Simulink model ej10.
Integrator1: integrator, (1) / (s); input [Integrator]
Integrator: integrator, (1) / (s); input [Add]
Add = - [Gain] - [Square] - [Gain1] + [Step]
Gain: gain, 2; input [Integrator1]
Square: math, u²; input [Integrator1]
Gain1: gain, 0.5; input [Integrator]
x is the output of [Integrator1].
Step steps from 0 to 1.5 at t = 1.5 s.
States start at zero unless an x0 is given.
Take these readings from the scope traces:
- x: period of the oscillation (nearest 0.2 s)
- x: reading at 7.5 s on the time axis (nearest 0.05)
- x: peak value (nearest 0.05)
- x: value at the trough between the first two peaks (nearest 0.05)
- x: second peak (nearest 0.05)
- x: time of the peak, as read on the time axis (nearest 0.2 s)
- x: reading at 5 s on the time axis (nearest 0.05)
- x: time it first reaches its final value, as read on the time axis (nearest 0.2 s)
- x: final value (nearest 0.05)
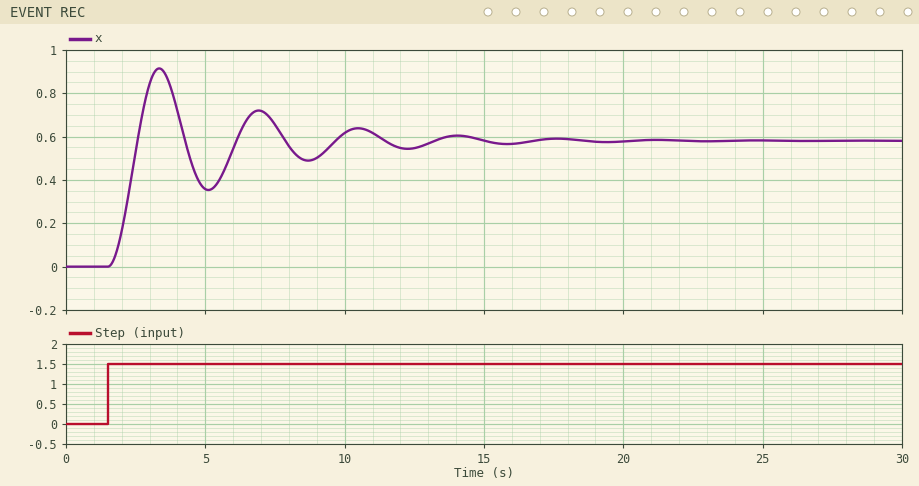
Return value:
3.6 s
0.65
0.90
0.35
0.70
3.4 s
0.35
2.6 s
0.60
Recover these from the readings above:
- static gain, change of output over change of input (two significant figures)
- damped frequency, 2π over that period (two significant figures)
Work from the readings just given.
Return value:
0.40
1.7 rad/s
